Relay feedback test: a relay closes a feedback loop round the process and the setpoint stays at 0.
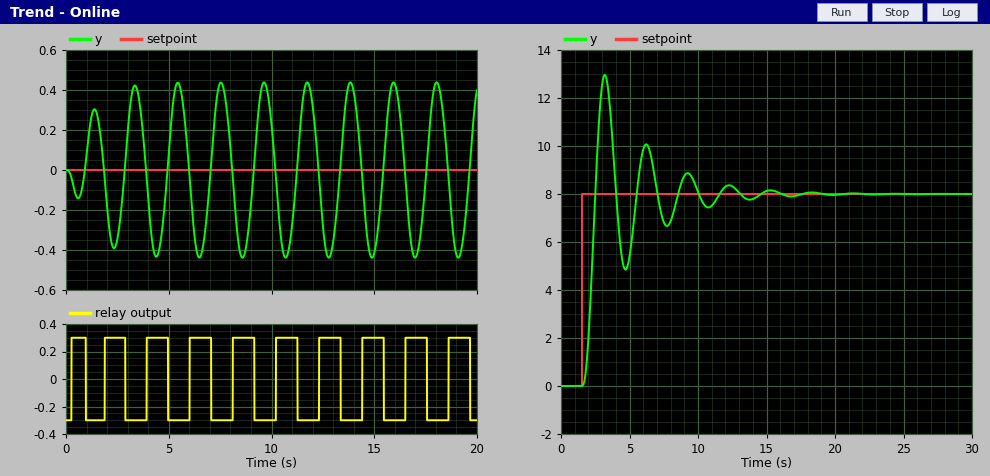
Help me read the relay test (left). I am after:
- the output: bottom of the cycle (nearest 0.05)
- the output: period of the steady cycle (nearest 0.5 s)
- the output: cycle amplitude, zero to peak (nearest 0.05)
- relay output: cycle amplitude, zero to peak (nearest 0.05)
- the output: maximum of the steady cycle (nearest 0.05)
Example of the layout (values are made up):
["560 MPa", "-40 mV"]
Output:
["-0.45", "2.0 s", "0.45", "0.30", "0.45"]
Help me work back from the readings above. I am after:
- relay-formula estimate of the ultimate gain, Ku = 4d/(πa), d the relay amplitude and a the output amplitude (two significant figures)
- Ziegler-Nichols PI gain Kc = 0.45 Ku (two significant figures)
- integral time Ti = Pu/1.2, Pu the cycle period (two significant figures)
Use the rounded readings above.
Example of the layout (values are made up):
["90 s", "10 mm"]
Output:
["0.85", "0.38", "1.7 s"]
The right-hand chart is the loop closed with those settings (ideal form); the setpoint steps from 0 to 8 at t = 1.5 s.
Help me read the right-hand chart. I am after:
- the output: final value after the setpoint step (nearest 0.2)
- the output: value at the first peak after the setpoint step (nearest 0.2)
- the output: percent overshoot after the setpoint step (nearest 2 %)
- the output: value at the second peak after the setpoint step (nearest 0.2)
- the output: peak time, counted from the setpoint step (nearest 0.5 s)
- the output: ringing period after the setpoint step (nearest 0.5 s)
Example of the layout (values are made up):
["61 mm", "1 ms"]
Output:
["8.0", "13.0", "62 %", "10.0", "1.5 s", "3.0 s"]
